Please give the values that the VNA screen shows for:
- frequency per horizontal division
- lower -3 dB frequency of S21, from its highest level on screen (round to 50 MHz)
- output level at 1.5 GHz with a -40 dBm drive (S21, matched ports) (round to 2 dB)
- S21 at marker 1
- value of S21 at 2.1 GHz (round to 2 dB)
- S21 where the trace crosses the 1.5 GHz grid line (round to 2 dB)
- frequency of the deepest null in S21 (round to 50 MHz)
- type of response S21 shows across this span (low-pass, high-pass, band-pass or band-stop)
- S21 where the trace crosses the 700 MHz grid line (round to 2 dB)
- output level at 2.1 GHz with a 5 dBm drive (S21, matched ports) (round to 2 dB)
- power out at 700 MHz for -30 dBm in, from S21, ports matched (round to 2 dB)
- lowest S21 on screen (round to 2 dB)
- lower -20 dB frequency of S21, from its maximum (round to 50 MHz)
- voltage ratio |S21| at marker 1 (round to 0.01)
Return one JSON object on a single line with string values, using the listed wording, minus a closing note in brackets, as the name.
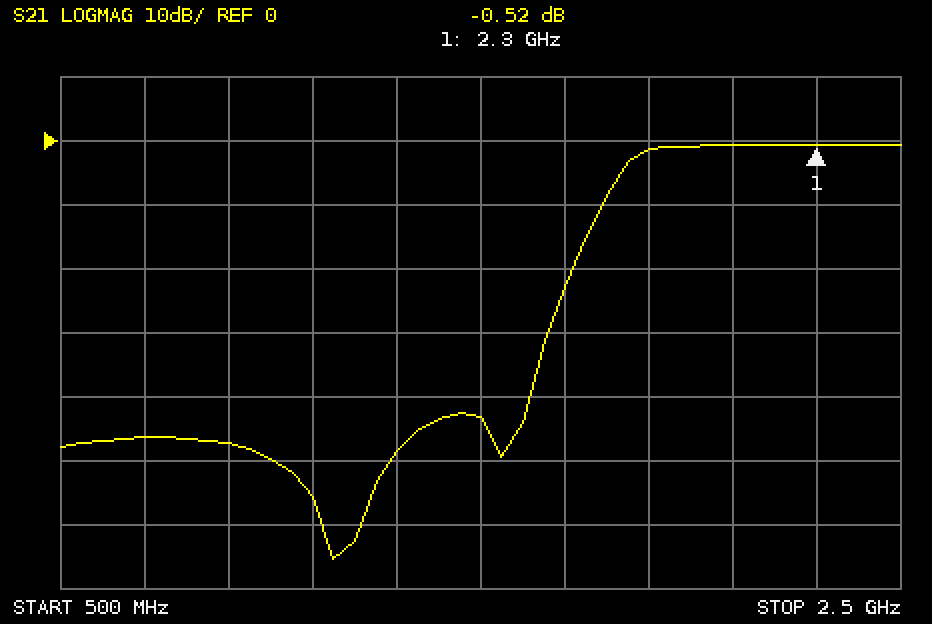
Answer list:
{"frequency per horizontal division": "200 MHz", "lower -3 dB frequency of S21, from its highest level on screen": "1.85 GHz", "output level at 1.5 GHz with a -40 dBm drive (S21, matched ports)": "-84 dBm", "S21 at marker 1": "-0.52 dB", "value of S21 at 2.1 GHz": "0 dB", "S21 where the trace crosses the 1.5 GHz grid line": "-44 dB", "frequency of the deepest null in S21": "1.15 GHz", "type of response S21 shows across this span": "high-pass", "S21 where the trace crosses the 700 MHz grid line": "-46 dB", "output level at 2.1 GHz with a 5 dBm drive (S21, matched ports)": "4 dBm", "power out at 700 MHz for -30 dBm in, from S21, ports matched": "-76 dBm", "lowest S21 on screen": "-66 dB", "lower -20 dB frequency of S21, from its maximum": "1.70 GHz", "voltage ratio |S21| at marker 1": "0.94"}
